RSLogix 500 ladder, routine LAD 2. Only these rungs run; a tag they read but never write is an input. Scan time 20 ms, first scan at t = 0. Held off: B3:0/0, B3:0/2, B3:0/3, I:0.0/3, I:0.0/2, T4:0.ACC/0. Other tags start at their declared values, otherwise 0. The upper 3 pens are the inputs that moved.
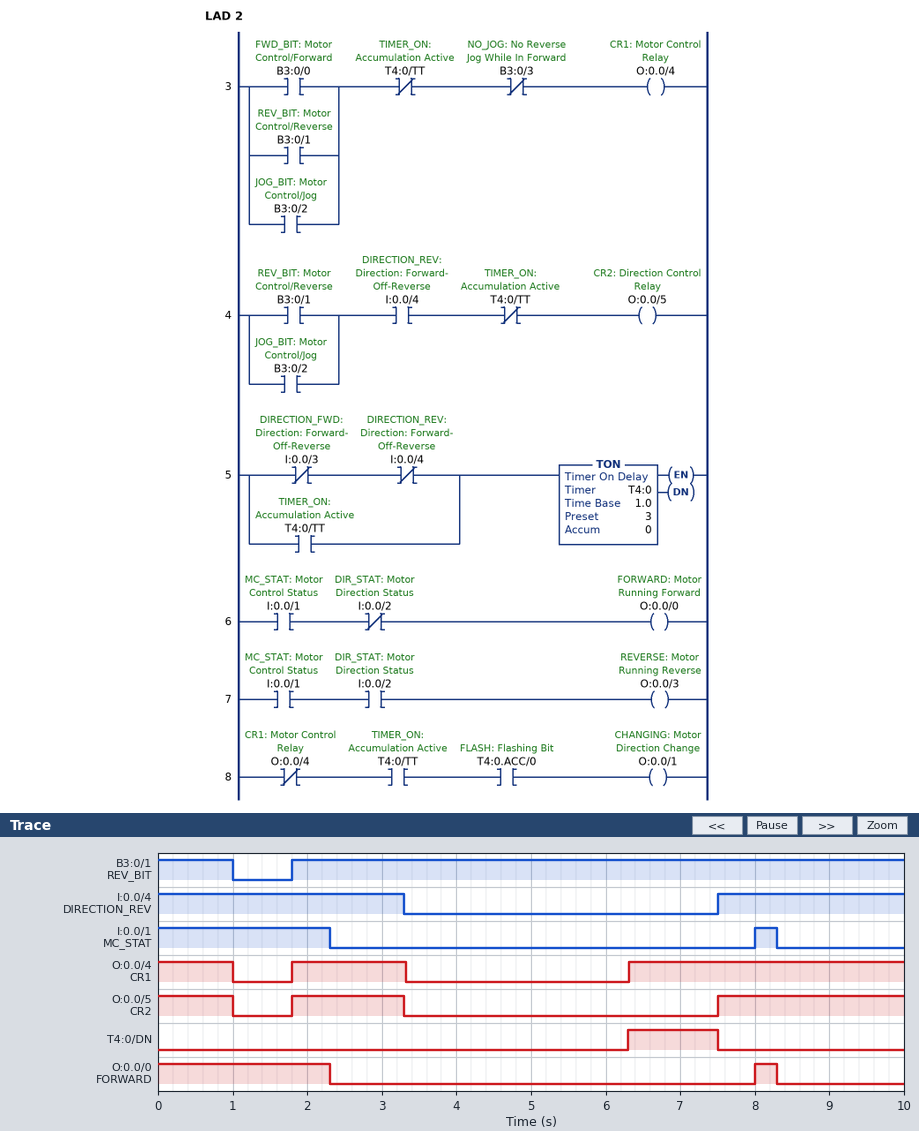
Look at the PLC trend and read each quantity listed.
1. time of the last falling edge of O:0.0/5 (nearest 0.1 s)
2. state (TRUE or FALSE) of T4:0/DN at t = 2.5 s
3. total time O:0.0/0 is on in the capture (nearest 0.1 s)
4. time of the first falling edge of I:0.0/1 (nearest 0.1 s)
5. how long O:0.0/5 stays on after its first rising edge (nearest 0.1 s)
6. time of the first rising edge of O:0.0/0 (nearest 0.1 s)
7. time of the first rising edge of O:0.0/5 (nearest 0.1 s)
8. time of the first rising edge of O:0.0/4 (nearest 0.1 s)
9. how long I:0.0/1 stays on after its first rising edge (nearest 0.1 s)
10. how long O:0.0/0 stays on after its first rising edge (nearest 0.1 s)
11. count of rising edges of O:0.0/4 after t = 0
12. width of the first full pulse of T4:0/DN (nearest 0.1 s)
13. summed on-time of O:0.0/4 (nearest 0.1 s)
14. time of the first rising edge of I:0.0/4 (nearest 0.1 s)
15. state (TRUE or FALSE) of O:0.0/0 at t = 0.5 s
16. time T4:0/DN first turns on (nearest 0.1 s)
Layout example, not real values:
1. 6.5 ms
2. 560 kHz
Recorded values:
1. 3.3 s
2. FALSE
3. 2.6 s
4. 2.3 s
5. 1.5 s
6. 8.0 s
7. 1.8 s
8. 1.8 s
9. 0.3 s
10. 0.3 s
11. 2
12. 1.2 s
13. 6.2 s
14. 7.5 s
15. TRUE
16. 6.3 s
